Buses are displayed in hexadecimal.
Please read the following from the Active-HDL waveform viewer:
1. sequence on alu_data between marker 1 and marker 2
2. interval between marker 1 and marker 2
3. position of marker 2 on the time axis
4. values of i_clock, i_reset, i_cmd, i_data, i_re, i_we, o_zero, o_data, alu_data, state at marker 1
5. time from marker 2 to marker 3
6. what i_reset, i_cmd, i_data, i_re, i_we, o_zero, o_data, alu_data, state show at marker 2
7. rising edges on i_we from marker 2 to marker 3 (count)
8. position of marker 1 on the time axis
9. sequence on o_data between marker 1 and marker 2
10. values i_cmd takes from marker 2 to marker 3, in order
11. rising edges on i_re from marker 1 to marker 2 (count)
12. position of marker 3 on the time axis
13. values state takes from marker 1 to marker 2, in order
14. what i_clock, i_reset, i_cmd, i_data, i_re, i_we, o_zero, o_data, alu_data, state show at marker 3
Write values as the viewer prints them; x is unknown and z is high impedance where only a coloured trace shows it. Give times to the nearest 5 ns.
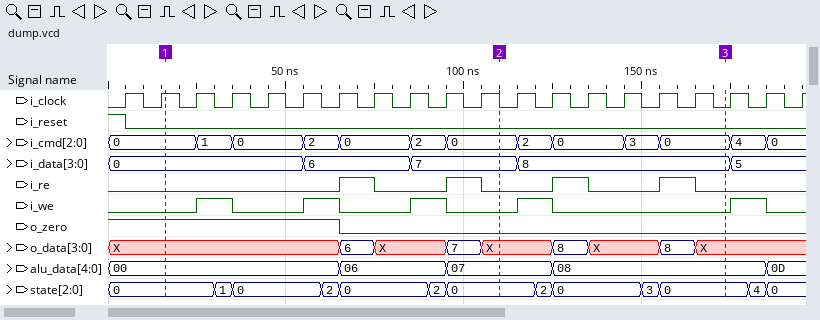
00, 06, 07
95 ns
110 ns
i_clock=1, i_reset=0, i_cmd=0, i_data=0, i_re=0, i_we=0, o_zero=1, o_data=X, alu_data=00, state=0
65 ns
i_reset=0, i_cmd=0, i_data=7, i_re=0, i_we=0, o_zero=0, o_data=X, alu_data=07, state=0
1
15 ns
X, 6, X, 7, X
0, 2, 0, 3, 0
2
175 ns
0, 1, 0, 2, 0, 2, 0
i_clock=0, i_reset=0, i_cmd=0, i_data=8, i_re=0, i_we=0, o_zero=0, o_data=X, alu_data=08, state=0
